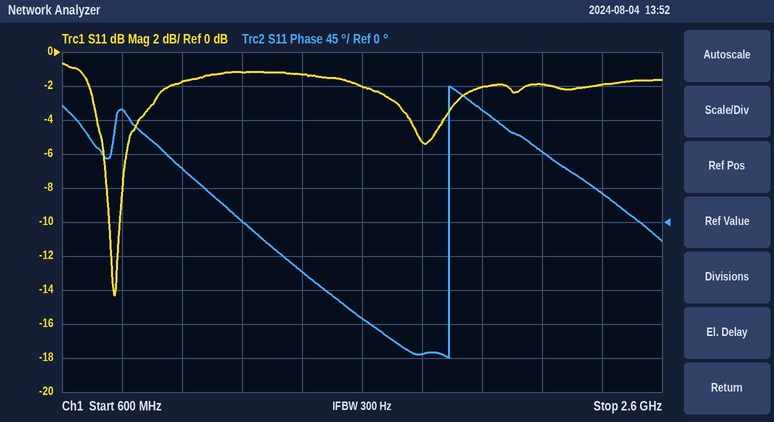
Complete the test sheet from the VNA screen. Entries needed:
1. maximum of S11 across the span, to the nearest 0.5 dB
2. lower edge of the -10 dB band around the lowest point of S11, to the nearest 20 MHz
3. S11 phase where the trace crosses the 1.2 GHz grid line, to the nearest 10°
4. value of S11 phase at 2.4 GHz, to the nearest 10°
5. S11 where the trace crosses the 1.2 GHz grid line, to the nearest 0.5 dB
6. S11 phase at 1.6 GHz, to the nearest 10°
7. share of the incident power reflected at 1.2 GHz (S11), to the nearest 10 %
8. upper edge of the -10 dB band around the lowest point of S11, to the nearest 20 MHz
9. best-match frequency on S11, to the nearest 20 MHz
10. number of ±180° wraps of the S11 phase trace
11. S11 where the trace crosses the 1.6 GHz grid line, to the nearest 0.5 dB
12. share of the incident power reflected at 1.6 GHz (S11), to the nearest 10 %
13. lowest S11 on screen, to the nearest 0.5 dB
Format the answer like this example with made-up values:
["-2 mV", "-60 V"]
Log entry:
["-0.5 dB", "760 MHz", "0°", "40°", "-1.0 dB", "-130°", "80 %", "800 MHz", "780 MHz", "1", "-2.0 dB", "60 %", "-14.5 dB"]
